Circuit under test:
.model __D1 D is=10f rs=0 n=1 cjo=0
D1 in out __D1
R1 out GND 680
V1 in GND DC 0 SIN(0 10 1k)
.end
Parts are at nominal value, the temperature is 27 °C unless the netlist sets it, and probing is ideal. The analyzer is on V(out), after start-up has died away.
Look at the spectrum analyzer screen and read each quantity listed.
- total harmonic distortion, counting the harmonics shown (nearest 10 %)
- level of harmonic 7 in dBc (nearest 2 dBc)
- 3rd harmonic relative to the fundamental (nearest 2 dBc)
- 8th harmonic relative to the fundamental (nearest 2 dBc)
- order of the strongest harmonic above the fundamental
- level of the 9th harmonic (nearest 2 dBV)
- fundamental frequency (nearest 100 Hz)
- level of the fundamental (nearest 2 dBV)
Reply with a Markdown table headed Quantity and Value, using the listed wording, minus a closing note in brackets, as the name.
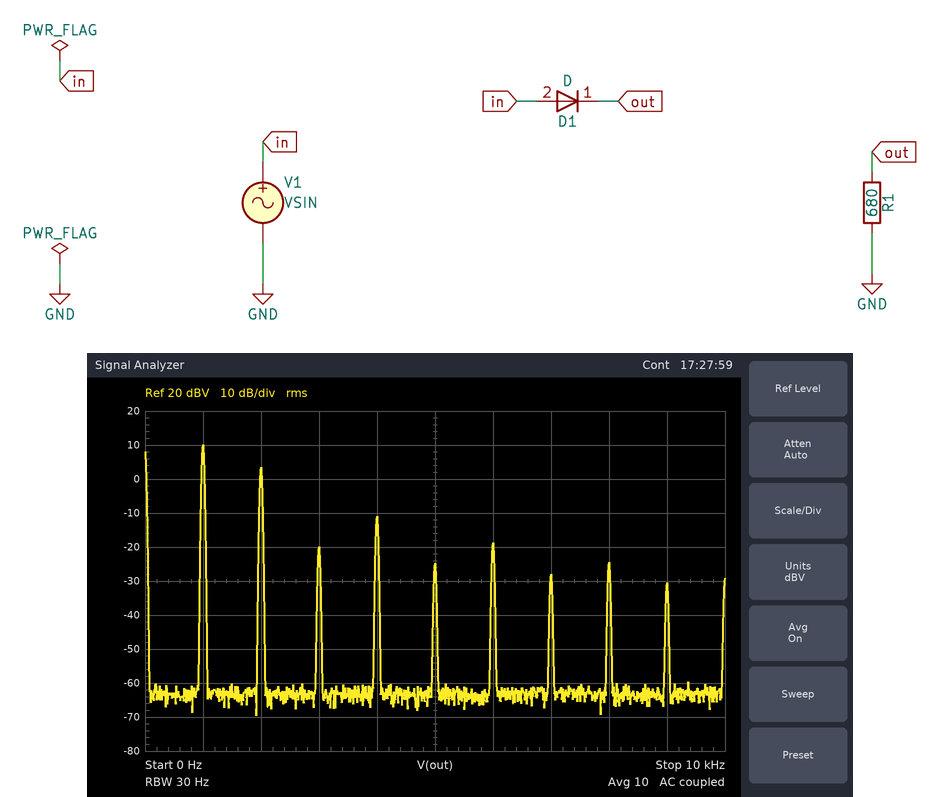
| Quantity | Value |
|---|---|
| total harmonic distortion, counting the harmonics shown | 50 % |
| level of harmonic 7 in dBc | -38 dBc |
| 3rd harmonic relative to the fundamental | -30 dBc |
| 8th harmonic relative to the fundamental | -34 dBc |
| order of the strongest harmonic above the fundamental | 2 |
| level of the 9th harmonic | -30 dBV |
| fundamental frequency | 1.0 kHz |
| level of the fundamental | 10 dBV |
